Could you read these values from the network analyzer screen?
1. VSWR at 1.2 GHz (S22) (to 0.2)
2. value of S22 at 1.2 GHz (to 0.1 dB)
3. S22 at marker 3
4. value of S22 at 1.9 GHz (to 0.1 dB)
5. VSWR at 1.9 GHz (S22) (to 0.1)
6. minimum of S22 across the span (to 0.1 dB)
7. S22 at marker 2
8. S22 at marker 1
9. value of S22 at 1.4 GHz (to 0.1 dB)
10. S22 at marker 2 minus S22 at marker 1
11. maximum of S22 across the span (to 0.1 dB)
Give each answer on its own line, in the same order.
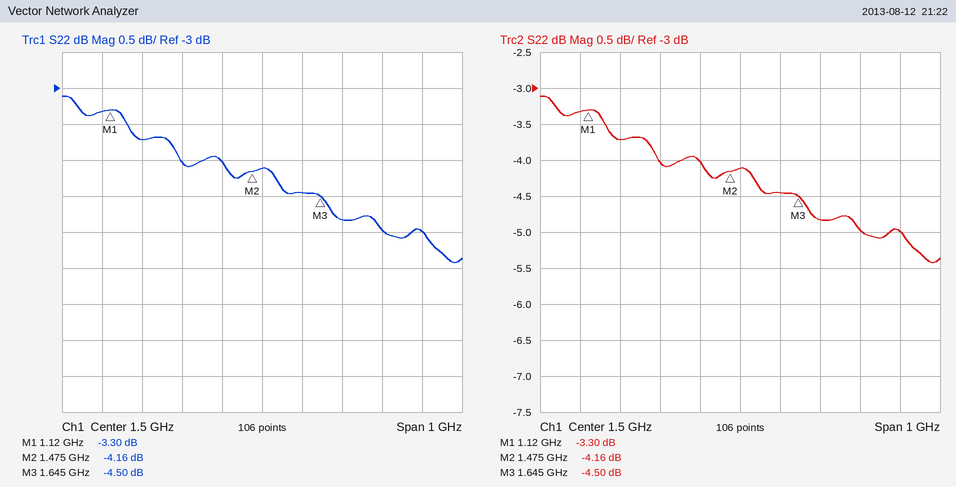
4.8
-3.7 dB
-4.50 dB
-5.0 dB
3.6
-5.4 dB
-4.16 dB
-3.30 dB
-4.0 dB
-0.86 dB
-3.1 dB
